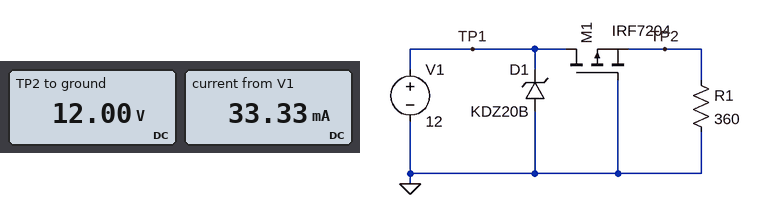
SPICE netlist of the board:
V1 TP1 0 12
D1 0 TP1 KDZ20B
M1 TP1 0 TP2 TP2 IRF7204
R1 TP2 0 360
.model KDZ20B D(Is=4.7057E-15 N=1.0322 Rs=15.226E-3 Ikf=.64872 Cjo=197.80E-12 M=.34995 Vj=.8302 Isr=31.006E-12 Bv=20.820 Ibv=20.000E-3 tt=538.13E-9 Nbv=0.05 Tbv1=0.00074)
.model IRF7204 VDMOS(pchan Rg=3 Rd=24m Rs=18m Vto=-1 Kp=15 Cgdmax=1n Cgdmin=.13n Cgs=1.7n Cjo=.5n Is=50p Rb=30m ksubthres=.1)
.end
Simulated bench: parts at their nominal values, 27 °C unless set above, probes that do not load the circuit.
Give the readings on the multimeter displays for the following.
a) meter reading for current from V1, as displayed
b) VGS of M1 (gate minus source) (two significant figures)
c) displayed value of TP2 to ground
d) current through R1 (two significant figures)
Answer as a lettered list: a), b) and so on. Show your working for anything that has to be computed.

a) 33.33 mA
b) 0 V - 12 V = -12 V
c) 12.00 V
d) (12 V) / 360 Ω = 33 mA
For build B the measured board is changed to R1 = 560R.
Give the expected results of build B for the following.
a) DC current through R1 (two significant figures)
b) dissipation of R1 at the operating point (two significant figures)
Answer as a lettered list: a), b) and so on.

a) 21 mA
b) 260 mW
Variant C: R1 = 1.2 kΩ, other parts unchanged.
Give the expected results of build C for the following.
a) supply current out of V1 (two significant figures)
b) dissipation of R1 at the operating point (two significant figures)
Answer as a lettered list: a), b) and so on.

a) 10 mA
b) 120 mW
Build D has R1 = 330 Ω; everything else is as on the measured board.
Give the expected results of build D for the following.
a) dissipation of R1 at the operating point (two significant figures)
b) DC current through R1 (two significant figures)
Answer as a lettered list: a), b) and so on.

a) 440 mW
b) 36 mA
